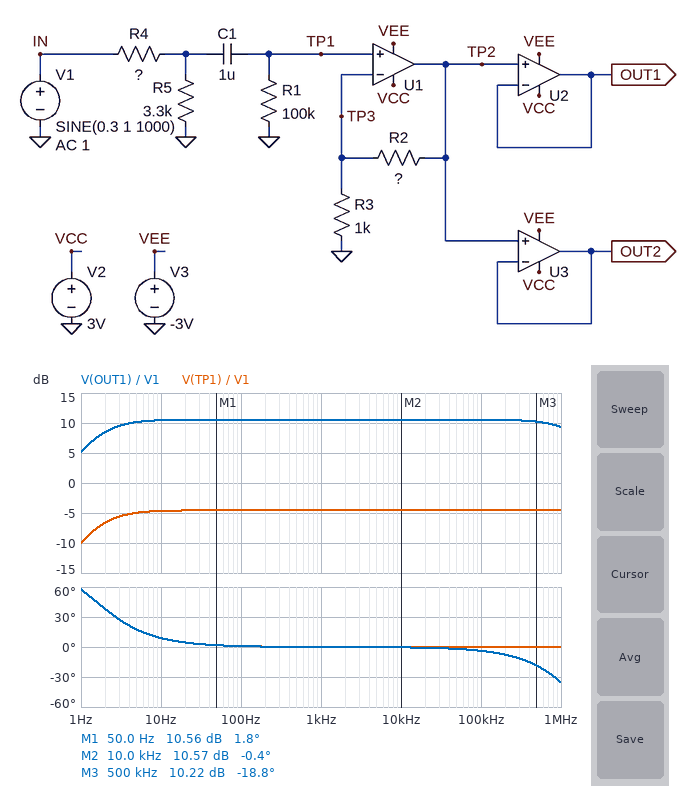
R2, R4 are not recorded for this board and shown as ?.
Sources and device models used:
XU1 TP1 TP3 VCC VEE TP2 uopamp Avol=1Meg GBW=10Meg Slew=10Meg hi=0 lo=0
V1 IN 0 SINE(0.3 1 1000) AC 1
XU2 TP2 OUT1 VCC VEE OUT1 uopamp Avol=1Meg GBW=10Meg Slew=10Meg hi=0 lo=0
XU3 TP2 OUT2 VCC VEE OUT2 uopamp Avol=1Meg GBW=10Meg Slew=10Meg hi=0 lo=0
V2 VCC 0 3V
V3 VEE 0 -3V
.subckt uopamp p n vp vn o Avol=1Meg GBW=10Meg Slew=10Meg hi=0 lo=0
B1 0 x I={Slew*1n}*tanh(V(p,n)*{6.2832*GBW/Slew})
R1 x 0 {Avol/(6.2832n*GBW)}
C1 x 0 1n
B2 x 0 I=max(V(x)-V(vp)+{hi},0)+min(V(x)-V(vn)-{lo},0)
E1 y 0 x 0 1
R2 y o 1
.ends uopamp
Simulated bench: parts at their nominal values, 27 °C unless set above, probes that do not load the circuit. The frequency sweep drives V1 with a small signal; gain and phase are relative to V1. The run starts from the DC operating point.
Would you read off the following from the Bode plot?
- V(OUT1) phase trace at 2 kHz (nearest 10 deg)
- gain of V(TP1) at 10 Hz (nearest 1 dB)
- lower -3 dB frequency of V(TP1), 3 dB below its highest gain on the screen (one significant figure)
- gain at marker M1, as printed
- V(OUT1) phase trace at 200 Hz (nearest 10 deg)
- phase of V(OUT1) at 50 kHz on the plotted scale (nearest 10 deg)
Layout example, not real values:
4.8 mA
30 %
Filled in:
0 deg
-5 dB
2 Hz
10.56 dB
0 deg
0 deg
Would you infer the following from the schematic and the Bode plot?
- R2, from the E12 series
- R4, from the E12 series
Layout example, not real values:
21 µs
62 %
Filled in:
4.7 kΩ
2.2 kΩ
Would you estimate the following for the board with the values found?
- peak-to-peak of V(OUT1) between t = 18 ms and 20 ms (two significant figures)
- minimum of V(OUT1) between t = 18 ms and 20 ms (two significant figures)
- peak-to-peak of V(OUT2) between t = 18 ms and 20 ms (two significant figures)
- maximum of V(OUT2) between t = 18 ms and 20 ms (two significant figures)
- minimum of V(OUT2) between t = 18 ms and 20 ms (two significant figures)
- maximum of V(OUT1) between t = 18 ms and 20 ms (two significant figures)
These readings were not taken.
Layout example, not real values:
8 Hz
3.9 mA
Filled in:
6.0 V
-3.0 V
6.0 V
3.0 V
-3.0 V
3.0 V
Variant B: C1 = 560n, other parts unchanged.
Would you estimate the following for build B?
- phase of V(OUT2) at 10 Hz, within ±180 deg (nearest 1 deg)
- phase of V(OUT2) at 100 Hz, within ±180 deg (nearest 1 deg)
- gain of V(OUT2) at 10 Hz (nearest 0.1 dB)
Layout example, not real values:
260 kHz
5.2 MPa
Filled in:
16 deg
2 deg
10.2 dB
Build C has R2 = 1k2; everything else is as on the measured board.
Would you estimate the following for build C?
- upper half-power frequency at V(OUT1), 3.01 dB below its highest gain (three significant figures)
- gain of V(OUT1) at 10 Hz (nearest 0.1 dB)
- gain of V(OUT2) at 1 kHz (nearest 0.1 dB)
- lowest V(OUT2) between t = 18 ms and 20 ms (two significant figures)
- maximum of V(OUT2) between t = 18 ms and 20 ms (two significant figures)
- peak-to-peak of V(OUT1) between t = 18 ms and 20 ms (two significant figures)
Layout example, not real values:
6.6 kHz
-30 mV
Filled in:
3.90 MHz
2.2 dB
2.3 dB
-1.3 V
1.3 V
2.6 V
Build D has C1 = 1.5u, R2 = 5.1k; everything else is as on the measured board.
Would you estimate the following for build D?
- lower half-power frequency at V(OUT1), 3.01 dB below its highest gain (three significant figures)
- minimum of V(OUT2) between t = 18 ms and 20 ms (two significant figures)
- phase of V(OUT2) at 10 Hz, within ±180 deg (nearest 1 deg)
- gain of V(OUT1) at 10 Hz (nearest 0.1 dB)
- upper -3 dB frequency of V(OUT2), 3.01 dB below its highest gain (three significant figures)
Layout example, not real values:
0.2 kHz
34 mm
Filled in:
1.05 Hz
-3.0 V
6 deg
11.1 dB
1.60 MHz
